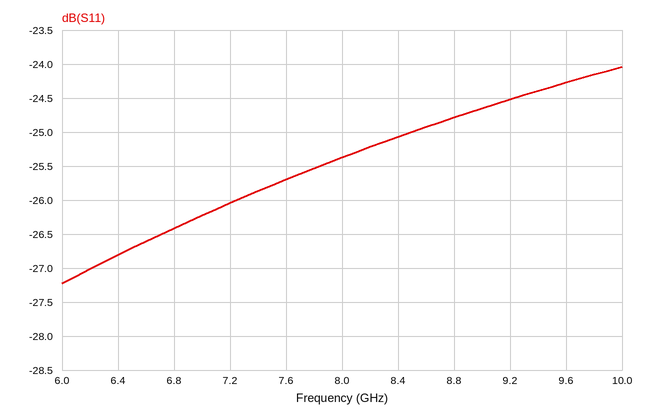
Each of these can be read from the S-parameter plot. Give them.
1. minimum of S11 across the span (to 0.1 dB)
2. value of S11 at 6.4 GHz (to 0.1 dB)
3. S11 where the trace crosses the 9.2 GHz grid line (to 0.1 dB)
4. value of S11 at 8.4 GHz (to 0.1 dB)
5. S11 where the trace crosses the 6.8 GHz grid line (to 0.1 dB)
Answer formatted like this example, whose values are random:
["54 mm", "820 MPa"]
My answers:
["-27.2 dB", "-26.8 dB", "-24.5 dB", "-25.1 dB", "-26.4 dB"]
